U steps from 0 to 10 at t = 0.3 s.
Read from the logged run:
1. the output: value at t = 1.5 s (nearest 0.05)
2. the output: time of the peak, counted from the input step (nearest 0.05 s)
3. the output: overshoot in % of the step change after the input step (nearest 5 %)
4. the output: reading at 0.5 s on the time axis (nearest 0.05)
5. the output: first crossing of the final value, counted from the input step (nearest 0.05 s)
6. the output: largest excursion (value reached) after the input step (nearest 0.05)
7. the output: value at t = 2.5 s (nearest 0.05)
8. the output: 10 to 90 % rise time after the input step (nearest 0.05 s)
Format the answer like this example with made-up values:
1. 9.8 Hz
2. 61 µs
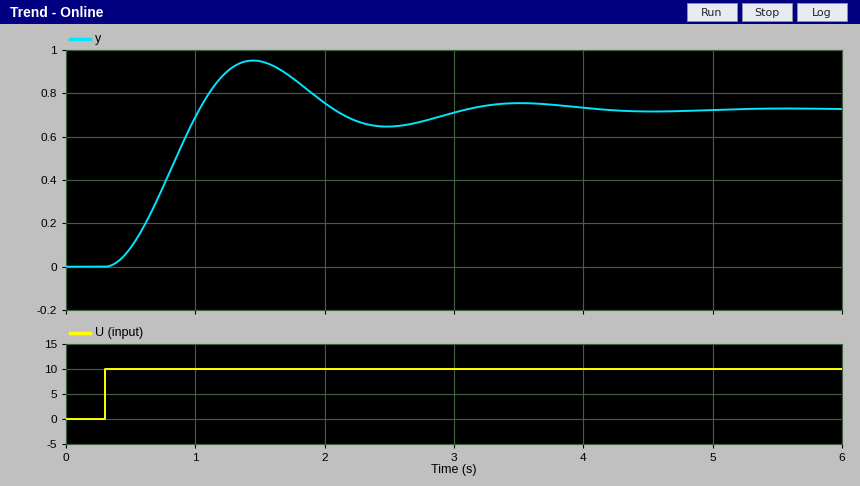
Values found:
1. 0.95
2. 1.15 s
3. 30 %
4. 0.10
5. 0.75 s
6. 0.95
7. 0.65
8. 0.50 s
